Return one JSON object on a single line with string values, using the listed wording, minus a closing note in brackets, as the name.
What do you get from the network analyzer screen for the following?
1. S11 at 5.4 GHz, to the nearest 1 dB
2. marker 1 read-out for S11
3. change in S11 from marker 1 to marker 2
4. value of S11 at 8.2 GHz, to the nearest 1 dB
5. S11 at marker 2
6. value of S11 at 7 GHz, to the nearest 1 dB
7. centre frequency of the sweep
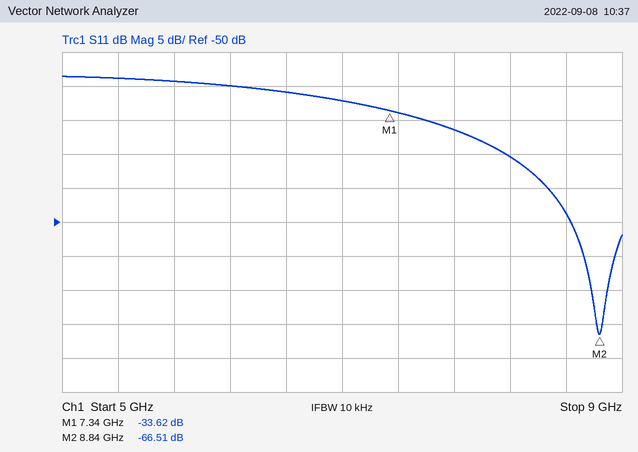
{"S11 at 5.4 GHz, to the nearest 1 dB": "-29 dB", "marker 1 read-out for S11": "-33.62 dB", "change in S11 from marker 1 to marker 2": "-32.89 dB", "value of S11 at 8.2 GHz, to the nearest 1 dB": "-40 dB", "S11 at marker 2": "-66.51 dB", "value of S11 at 7 GHz, to the nearest 1 dB": "-32 dB", "centre frequency of the sweep": "7 GHz"}
